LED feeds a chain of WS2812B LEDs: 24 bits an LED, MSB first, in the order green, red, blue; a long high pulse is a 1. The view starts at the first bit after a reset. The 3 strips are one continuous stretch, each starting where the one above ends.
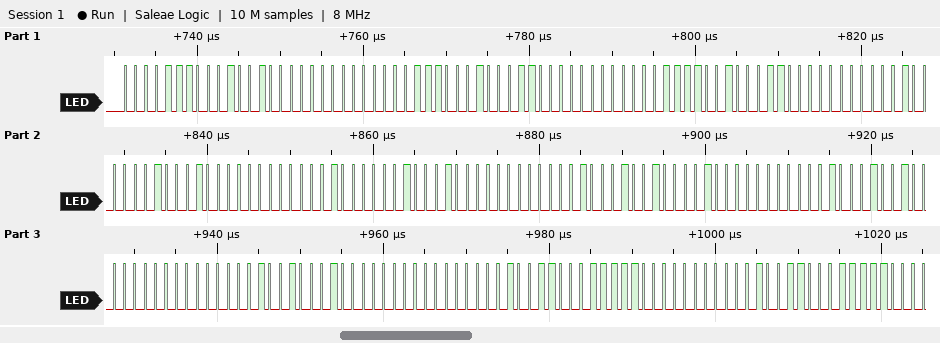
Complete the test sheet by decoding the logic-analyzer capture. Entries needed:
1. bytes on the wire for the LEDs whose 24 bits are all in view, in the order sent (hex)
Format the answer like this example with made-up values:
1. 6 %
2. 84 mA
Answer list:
1. 0E 24 00 0E 23 00 0F 23 00 10 22 00 10 22 00 11 21 00 11 20 00 12 20 00 13 1F 00
